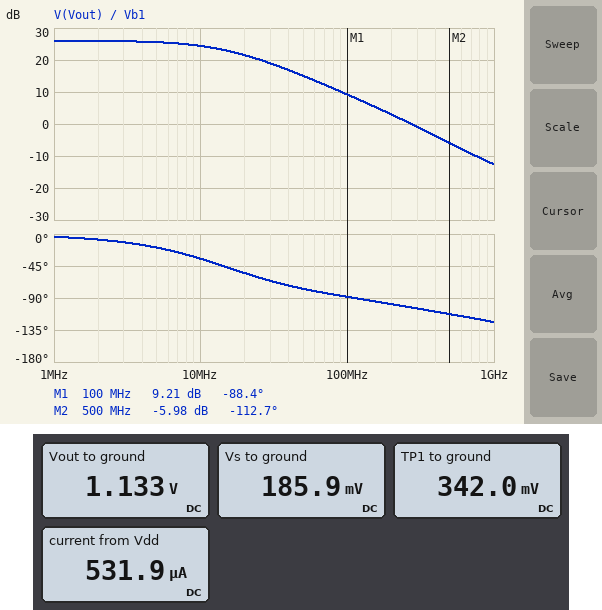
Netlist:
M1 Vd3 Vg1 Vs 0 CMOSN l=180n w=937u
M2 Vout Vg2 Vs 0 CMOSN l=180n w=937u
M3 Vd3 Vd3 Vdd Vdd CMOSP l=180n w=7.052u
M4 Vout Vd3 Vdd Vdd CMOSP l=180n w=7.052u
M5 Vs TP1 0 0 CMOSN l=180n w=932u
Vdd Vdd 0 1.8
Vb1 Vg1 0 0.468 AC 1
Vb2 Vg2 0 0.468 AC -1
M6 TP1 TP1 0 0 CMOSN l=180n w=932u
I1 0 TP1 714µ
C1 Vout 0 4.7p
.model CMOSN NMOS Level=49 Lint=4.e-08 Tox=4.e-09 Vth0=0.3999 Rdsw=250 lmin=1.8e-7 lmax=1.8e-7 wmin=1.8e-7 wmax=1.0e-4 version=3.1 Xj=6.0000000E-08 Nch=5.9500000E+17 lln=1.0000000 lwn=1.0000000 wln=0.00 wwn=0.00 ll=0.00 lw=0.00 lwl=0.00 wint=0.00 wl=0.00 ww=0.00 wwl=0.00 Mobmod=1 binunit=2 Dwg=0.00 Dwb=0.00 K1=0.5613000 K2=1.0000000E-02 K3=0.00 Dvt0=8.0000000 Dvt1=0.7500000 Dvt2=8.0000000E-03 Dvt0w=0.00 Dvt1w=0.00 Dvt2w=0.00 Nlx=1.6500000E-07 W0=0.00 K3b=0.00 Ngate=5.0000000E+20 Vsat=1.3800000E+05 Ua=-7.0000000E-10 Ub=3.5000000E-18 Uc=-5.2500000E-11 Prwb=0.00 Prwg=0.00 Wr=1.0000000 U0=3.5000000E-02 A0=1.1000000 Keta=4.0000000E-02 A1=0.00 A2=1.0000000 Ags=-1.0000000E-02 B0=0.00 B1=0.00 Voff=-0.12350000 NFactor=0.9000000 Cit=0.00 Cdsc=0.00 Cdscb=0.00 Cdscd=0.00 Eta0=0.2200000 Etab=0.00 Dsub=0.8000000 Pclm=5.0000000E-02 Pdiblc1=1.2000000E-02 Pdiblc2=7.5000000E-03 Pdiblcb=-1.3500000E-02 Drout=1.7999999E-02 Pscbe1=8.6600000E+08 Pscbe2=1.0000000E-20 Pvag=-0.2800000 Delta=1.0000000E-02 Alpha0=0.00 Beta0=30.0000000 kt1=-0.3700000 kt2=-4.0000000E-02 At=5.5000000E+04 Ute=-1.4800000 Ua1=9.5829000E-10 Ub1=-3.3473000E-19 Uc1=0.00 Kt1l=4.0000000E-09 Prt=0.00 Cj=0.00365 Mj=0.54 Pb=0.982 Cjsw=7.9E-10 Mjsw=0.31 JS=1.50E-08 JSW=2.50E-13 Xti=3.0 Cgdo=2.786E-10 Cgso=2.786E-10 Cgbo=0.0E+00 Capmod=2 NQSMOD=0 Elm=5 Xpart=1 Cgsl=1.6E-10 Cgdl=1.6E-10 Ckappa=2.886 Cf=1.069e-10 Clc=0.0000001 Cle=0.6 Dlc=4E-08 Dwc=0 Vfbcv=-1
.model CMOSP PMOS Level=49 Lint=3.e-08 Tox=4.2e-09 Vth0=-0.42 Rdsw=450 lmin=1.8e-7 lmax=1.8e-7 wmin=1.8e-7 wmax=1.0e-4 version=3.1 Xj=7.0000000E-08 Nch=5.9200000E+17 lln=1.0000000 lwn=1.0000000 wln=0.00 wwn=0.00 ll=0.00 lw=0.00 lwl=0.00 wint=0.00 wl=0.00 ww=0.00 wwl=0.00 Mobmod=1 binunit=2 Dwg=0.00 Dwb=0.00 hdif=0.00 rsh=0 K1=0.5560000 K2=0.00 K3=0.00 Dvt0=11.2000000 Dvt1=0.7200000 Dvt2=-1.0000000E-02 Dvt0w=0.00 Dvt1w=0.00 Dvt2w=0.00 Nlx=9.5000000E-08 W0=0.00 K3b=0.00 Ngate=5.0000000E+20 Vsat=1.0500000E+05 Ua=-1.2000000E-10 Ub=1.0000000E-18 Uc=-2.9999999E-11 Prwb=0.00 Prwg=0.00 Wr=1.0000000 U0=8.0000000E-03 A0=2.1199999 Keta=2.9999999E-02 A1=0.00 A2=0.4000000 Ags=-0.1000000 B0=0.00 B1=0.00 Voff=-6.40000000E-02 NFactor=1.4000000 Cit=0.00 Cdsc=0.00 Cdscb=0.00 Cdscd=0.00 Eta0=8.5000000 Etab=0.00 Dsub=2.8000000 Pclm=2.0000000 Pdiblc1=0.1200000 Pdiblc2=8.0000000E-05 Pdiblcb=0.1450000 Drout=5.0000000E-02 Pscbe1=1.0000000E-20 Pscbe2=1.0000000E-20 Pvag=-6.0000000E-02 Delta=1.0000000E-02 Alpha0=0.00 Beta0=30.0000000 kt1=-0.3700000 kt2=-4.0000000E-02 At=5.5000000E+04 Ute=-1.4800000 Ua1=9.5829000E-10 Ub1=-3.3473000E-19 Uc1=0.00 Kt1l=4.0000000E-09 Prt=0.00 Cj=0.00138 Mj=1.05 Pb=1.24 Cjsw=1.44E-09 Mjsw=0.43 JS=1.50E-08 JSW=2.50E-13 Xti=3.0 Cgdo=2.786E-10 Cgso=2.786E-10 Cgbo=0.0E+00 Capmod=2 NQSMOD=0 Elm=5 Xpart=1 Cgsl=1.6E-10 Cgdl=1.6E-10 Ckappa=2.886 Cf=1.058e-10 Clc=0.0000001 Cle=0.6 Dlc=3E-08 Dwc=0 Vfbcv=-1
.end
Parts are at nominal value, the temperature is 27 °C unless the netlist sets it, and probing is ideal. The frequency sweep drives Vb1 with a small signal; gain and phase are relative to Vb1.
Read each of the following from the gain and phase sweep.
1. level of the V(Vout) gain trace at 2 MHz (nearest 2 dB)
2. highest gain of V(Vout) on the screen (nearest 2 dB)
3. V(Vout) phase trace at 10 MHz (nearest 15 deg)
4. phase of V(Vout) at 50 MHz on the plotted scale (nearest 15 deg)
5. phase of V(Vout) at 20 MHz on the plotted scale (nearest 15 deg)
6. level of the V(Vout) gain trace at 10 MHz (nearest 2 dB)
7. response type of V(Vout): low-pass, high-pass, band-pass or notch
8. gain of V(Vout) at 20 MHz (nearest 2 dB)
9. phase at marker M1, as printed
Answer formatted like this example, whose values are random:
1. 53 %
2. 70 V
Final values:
1. 26 dB
2. 26 dB
3. -30 deg
4. -75 deg
5. -60 deg
6. 24 dB
7. low-pass
8. 22 dB
9. -88.4 deg
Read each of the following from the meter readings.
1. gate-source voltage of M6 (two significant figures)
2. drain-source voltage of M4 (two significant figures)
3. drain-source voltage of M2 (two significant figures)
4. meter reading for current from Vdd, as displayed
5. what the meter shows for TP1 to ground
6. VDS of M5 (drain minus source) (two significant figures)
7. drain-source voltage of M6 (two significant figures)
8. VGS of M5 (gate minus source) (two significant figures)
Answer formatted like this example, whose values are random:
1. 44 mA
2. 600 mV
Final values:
1. 340 mV
2. -670 mV
3. 950 mV
4. 531.9 µA
5. 342.0 mV
6. 190 mV
7. 340 mV
8. 340 mV
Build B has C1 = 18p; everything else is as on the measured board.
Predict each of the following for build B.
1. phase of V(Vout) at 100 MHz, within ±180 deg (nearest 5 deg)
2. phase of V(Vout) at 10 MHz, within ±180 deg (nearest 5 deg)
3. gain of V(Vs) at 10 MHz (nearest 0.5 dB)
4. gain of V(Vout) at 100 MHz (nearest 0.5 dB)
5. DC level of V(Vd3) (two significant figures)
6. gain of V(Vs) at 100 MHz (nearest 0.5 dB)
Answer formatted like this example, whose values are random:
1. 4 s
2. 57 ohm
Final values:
1. -95 deg
2. -65 deg
3. -12.5 dB
4. -1.0 dB
5. 1.1 V
6. -18.5 dB
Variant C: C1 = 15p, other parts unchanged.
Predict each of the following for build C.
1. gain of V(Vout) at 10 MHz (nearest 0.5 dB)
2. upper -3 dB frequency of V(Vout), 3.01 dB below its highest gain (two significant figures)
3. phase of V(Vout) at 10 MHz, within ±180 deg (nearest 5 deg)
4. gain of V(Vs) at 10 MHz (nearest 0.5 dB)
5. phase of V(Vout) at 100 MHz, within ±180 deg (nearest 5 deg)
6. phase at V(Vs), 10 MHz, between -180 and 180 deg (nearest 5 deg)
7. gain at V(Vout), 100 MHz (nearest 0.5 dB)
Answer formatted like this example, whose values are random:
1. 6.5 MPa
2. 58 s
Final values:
1. 19.5 dB
2. 5.3 MHz
3. -65 deg
4. -11.5 dB
5. -95 deg
6. -90 deg
7. 0.5 dB
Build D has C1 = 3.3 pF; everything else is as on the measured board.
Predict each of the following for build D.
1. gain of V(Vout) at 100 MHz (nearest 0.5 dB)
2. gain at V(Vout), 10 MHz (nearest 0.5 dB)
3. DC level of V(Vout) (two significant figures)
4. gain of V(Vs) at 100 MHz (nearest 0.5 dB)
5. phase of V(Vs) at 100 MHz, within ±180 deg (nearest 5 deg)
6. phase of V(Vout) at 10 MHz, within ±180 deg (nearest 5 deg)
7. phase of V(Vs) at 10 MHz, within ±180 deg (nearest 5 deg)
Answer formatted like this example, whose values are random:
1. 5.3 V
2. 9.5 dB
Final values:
1. 11.5 dB
2. 25.0 dB
3. 1.1 V
4. -17.0 dB
5. -150 deg
6. -30 deg
7. -35 deg
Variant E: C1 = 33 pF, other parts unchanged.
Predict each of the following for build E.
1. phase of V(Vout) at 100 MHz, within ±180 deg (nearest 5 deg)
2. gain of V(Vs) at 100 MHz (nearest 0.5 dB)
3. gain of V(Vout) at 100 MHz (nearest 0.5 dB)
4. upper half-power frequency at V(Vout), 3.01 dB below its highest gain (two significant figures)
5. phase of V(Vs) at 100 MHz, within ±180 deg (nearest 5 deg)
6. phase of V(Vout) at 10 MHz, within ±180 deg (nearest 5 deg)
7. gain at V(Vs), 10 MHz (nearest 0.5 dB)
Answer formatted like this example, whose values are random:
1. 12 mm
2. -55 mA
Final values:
1. -95 deg
2. -18.5 dB
3. -6.0 dB
4. 2.5 MHz
5. 165 deg
6. -75 deg
7. -15.0 dB
